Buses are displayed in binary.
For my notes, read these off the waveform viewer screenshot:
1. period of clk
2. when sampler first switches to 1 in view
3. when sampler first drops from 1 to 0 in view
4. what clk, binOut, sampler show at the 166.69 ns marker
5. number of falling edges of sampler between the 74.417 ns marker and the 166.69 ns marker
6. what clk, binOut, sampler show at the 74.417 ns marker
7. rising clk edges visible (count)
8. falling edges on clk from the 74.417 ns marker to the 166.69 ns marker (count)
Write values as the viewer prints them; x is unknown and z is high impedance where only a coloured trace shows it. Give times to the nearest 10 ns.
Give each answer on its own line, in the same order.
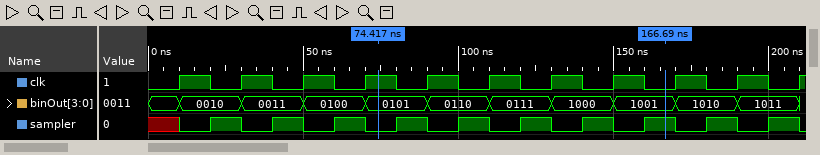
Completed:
20 ns
20 ns
30 ns
clk=0, binOut=1001, sampler=1
4
clk=1, binOut=0101, sampler=0
11
5
